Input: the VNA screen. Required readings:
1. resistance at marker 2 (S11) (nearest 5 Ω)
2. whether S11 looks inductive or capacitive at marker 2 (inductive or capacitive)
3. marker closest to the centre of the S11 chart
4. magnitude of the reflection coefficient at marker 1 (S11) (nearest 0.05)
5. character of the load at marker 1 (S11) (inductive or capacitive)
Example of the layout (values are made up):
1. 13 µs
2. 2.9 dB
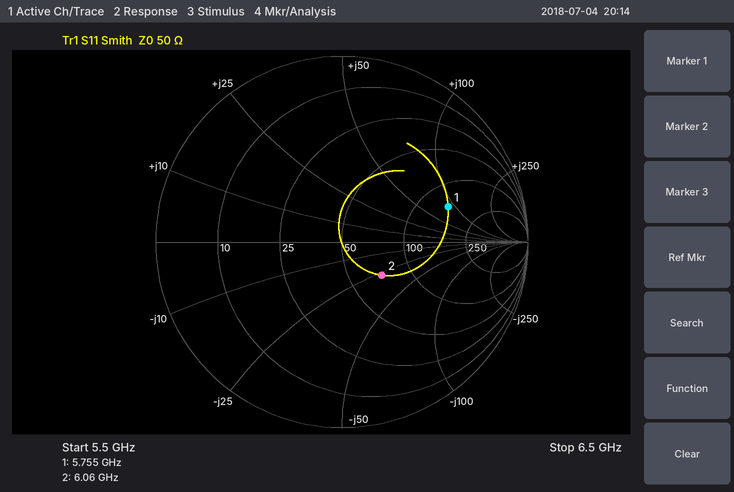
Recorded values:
1. 70 Ω
2. capacitive
3. marker 2
4. 0.60
5. inductive
